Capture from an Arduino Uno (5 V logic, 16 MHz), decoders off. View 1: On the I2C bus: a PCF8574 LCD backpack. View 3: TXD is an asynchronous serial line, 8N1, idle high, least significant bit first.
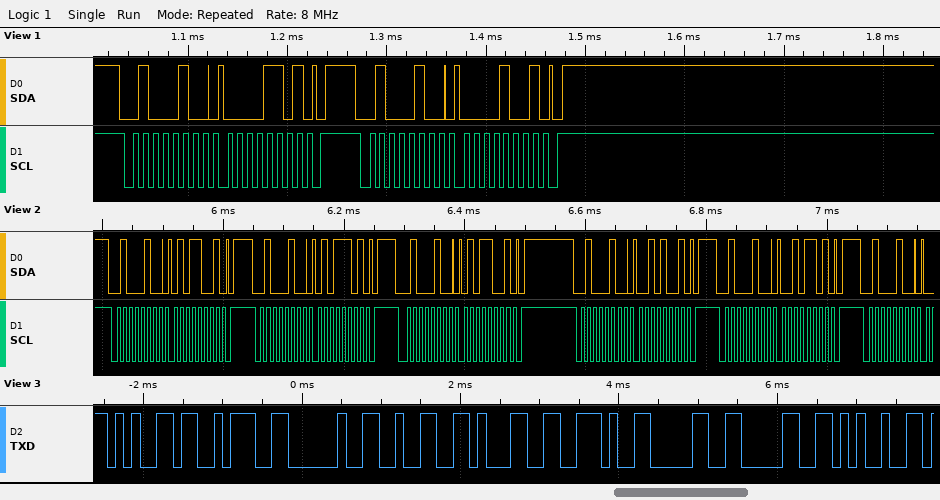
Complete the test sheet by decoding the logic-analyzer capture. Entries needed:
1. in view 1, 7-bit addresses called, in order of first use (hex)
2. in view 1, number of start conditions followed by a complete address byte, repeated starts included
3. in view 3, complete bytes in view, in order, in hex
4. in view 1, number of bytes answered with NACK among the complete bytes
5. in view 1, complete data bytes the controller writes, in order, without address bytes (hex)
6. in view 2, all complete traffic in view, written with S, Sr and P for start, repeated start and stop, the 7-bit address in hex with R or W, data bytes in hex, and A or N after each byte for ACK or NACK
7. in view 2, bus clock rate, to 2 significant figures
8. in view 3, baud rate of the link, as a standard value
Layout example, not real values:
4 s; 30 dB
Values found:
0x22; 2; 65 3A 20 32 31 2E 30 30 25; 0; 0D 09; S 22W A 59 A P S 22W A 5D A P S 22W A 59 A P S 22W A 29 A P S 22W A 2D A P S 22W A; 100 kHz; 9600 baud
